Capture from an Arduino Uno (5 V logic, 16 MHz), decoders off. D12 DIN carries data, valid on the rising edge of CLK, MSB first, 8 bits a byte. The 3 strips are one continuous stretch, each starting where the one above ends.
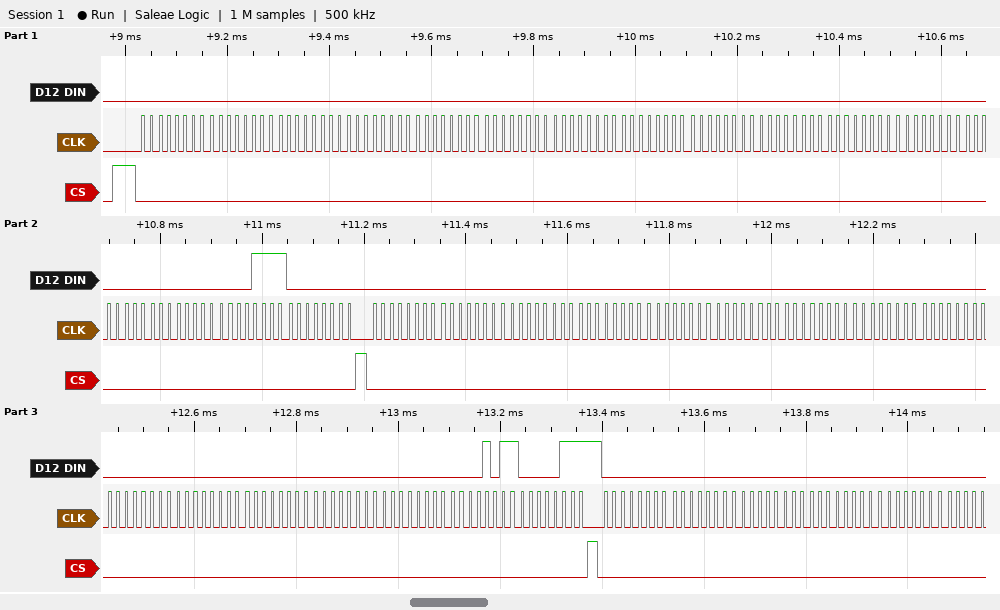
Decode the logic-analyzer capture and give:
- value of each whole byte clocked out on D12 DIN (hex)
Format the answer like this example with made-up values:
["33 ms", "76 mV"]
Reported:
["0x00 0x00 0x00 0x00 0x00 0x00 0x00 0x00 0x00 0x00 0x00 0x00 0x00 0x00 0x0F 0x00 0x00 0x00 0x00 0x00 0x00 0x00 0x00 0x00 0x00 0x00 0x00 0x00 0x00 0x00 0x0B 0x07 0x00 0x00 0x00 0x00 0x00"]
